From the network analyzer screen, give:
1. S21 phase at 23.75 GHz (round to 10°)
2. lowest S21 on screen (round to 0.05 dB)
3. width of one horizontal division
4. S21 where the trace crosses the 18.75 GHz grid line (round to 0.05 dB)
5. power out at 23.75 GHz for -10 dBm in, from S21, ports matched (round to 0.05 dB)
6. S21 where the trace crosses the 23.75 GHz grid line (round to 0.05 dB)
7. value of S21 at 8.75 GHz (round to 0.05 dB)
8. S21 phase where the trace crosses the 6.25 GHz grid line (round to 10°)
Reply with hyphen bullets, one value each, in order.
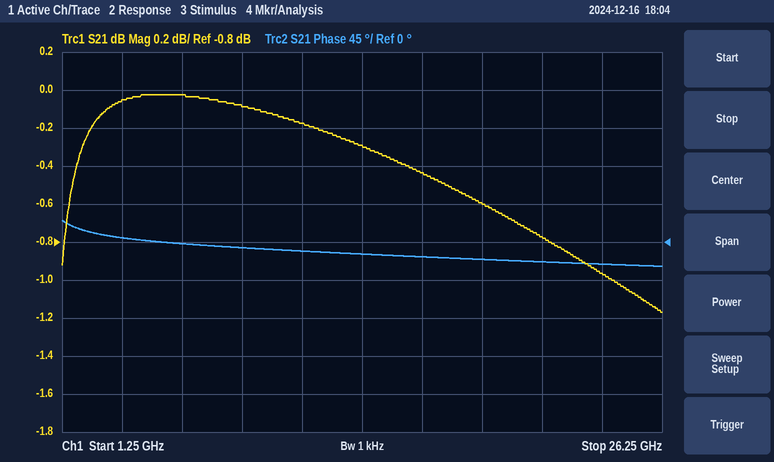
- -30°
- -1.15 dB
- 2.5 GHz
- -0.60 dB
- -10.95 dBm
- -0.95 dB
- -0.10 dB
- 0°
